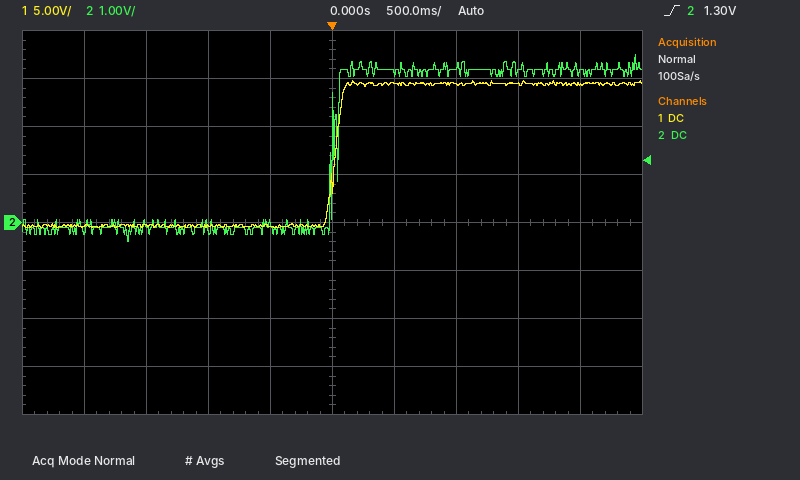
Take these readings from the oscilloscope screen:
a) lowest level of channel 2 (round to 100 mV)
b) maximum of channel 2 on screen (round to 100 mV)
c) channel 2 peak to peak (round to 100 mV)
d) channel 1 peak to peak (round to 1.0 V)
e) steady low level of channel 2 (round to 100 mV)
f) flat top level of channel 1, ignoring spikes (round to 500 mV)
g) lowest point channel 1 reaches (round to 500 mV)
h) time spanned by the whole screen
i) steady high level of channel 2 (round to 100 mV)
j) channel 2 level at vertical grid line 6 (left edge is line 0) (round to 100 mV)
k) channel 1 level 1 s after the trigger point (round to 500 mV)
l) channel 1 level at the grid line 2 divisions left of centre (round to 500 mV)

-400 mV
3.5 V
3.9 V
15.0 V
-100 mV
14.5 V
-500 mV
5 s
3.2 V
3.1 V
14.5 V
-500 mV
